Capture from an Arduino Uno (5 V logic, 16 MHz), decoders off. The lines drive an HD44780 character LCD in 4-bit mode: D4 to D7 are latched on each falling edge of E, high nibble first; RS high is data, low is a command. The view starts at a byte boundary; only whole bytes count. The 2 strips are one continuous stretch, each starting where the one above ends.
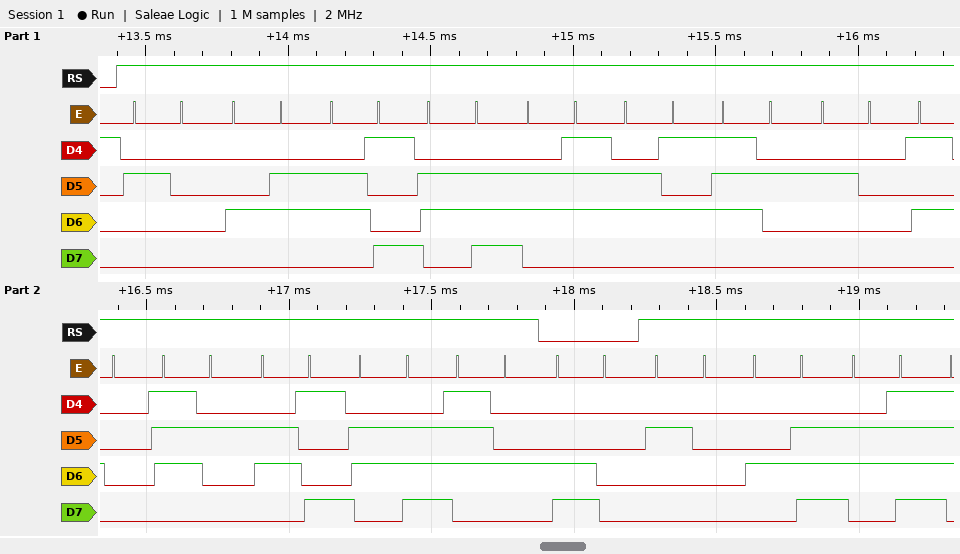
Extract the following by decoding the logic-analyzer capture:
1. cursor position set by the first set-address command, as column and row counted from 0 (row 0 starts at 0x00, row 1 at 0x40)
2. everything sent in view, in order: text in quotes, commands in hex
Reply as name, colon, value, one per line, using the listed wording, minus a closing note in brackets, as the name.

cursor position set by the first set-address command, as column and row counted from 0: column 0, row 1
everything sent in view, in order: text in quotes, commands in hex: " Finger Print" 0xC0 " No"
